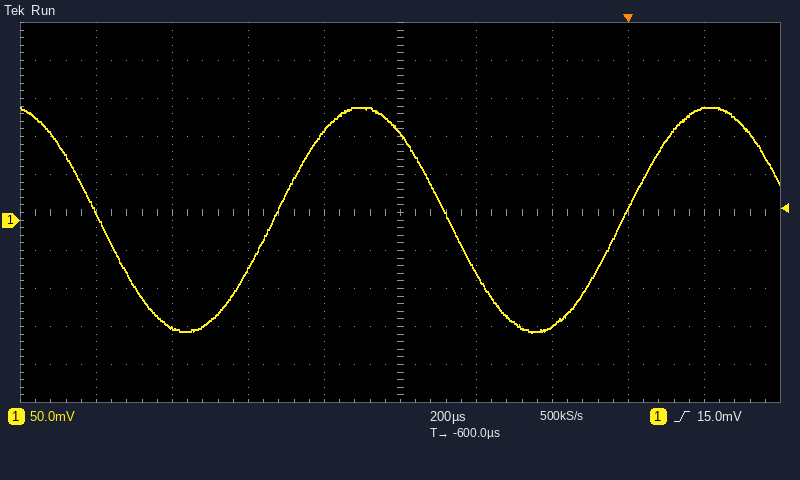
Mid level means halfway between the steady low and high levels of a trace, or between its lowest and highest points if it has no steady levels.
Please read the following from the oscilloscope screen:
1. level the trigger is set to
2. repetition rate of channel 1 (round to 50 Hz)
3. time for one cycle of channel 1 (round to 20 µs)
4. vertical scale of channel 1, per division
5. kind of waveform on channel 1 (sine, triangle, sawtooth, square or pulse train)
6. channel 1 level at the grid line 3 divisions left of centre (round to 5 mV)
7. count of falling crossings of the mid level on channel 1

15.0 mV
1.10 kHz
920 µs
50 mV
sine
-140 mV
2
